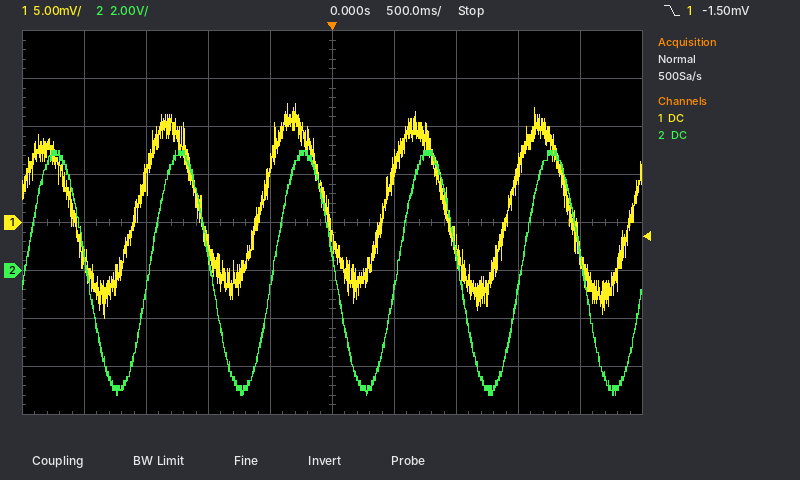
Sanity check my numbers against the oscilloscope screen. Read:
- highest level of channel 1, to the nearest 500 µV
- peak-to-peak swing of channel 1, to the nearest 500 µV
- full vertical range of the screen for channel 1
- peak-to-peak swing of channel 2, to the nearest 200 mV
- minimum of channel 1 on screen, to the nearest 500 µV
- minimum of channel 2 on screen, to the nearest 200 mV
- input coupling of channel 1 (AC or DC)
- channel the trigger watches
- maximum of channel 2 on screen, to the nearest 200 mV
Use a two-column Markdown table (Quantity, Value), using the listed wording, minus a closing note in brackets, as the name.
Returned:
| Quantity | Value |
|---|---|
| highest level of channel 1, to the nearest 500 µV | 12.5 mV |
| peak-to-peak swing of channel 1, to the nearest 500 µV | 22.5 mV |
| full vertical range of the screen for channel 1 | 40 mV |
| peak-to-peak swing of channel 2, to the nearest 200 mV | 10.2 V |
| minimum of channel 1 on screen, to the nearest 500 µV | -10.0 mV |
| minimum of channel 2 on screen, to the nearest 200 mV | -5.2 V |
| input coupling of channel 1 | DC |
| channel the trigger watches | channel 1 |
| maximum of channel 2 on screen, to the nearest 200 mV | 5.0 V |
